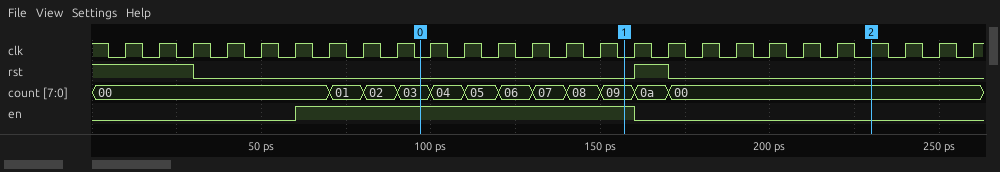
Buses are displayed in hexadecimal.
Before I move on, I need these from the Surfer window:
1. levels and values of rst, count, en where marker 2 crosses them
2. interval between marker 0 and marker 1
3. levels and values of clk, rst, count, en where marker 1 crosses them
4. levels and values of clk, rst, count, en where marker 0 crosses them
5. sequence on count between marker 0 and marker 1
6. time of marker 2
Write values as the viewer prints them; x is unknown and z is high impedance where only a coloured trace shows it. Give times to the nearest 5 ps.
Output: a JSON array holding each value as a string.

["rst=0, count=00, en=0", "60 ps", "clk=0, rst=0, count=09, en=1", "clk=0, rst=0, count=03, en=1", "03, 04, 05, 06, 07, 08, 09", "230 ps"]
